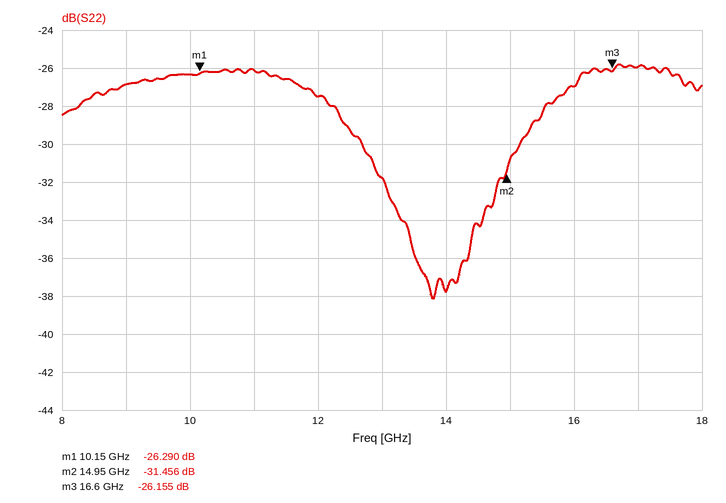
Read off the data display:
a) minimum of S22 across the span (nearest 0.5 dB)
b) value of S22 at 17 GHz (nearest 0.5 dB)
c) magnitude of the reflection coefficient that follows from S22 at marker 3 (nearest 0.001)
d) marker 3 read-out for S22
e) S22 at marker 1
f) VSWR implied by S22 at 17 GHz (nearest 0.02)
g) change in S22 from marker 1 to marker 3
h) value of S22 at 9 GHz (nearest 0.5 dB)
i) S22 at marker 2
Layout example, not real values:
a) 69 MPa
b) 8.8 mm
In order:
a) -38.0 dB
b) -26.0 dB
c) 0.049
d) -26.155 dB
e) -26.290 dB
f) 1.10
g) 0.135 dB
h) -27.0 dB
i) -31.456 dB
